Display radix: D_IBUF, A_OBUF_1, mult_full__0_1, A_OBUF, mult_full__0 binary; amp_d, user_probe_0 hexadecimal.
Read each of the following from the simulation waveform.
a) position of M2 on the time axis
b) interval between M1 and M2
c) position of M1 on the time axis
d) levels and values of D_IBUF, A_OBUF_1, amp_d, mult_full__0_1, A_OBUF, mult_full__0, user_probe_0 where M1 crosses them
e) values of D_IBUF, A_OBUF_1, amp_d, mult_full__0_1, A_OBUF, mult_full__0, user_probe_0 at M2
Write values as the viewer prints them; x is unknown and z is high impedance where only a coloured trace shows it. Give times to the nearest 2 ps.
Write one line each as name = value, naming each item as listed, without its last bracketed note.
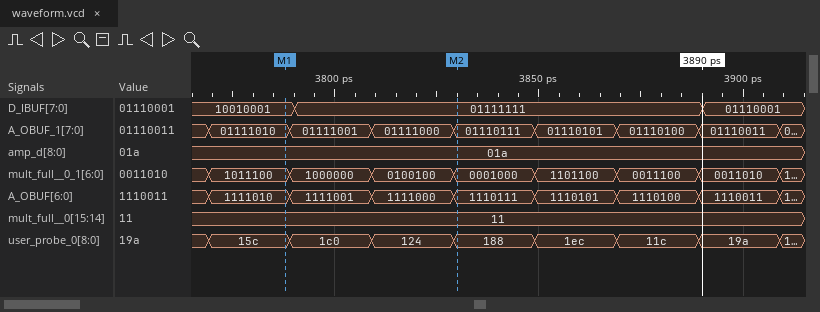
position of M2 on the time axis = 3830 ps
interval between M1 and M2 = 42 ps
position of M1 on the time axis = 3788 ps
levels and values of D_IBUF, A_OBUF_1, amp_d, mult_full__0_1, A_OBUF, mult_full__0, user_probe_0 where M1 crosses them = D_IBUF=10010001, A_OBUF_1=01111010, amp_d=01a, mult_full__0_1=1011100, A_OBUF=1111010, mult_full__0=11, user_probe_0=15c
values of D_IBUF, A_OBUF_1, amp_d, mult_full__0_1, A_OBUF, mult_full__0, user_probe_0 at M2 = D_IBUF=01111111, A_OBUF_1=01110111, amp_d=01a, mult_full__0_1=0001000, A_OBUF=1110111, mult_full__0=11, user_probe_0=188
